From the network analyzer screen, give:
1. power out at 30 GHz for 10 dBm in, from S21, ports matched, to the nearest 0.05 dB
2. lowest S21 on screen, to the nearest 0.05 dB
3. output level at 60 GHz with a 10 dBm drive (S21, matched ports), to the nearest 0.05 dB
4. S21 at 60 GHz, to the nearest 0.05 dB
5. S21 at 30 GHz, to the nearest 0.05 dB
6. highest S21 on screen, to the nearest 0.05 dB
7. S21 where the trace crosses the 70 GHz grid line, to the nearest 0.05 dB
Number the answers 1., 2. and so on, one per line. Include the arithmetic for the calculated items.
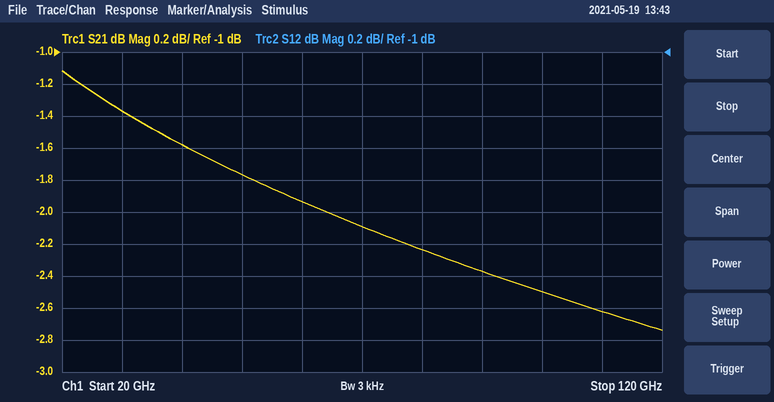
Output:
1. 10 dBm + (-1.35 dB) = 8.65 dBm
2. -2.75 dB
3. 10 dBm + (-1.95 dB) = 8.05 dBm
4. -1.95 dB
5. -1.35 dB
6. -1.10 dB
7. -2.10 dB
